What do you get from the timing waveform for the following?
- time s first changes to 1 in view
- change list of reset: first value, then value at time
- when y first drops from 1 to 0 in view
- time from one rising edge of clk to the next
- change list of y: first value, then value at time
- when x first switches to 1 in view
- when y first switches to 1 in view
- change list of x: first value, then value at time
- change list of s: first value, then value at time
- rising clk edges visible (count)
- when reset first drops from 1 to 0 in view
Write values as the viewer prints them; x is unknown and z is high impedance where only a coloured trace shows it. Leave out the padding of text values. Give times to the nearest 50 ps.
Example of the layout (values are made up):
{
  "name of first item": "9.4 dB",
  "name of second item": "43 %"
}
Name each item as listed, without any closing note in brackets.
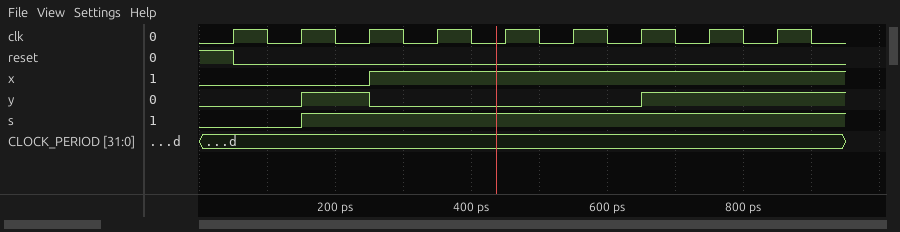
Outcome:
{
  "time s first changes to 1 in view": "150 ps",
  "change list of reset: first value, then value at time": "1, 0 at 50 ps",
  "when y first drops from 1 to 0 in view": "250 ps",
  "time from one rising edge of clk to the next": "100 ps",
  "change list of y: first value, then value at time": "0, 1 at 150 ps, 0 at 250 ps, 1 at 650 ps",
  "when x first switches to 1 in view": "250 ps",
  "when y first switches to 1 in view": "150 ps",
  "change list of x: first value, then value at time": "0, 1 at 250 ps",
  "change list of s: first value, then value at time": "0, 1 at 150 ps",
  "rising clk edges visible": "9",
  "when reset first drops from 1 to 0 in view": "50 ps"
}
